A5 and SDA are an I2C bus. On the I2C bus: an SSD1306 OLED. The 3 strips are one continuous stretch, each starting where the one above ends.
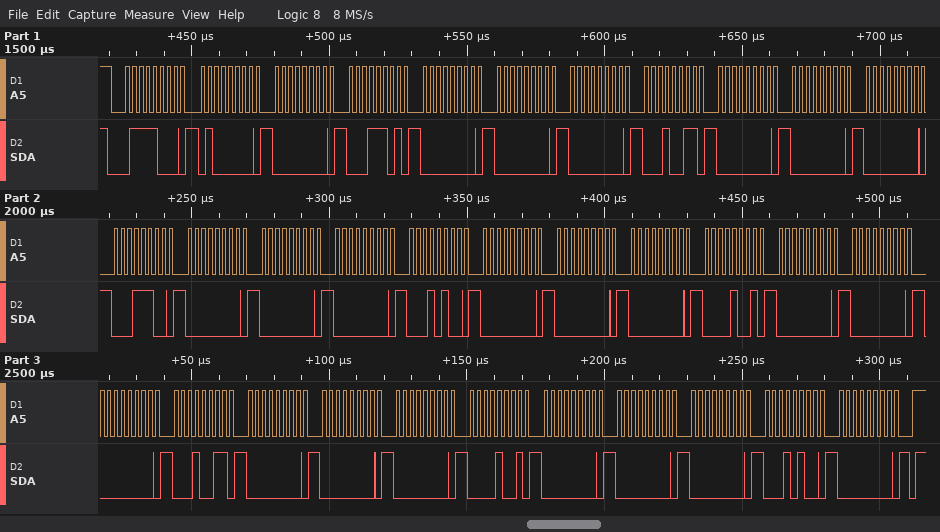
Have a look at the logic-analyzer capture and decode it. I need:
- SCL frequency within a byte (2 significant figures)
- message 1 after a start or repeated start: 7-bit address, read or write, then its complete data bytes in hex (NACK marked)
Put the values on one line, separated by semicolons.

400 kHz; 0x3C write: 40 00 1D 00 00 00 13 00 00 00 1C 00 00 00 14 00 00 00 09 00 00 00 13 00 00 00 09 00 00 00 14 00
